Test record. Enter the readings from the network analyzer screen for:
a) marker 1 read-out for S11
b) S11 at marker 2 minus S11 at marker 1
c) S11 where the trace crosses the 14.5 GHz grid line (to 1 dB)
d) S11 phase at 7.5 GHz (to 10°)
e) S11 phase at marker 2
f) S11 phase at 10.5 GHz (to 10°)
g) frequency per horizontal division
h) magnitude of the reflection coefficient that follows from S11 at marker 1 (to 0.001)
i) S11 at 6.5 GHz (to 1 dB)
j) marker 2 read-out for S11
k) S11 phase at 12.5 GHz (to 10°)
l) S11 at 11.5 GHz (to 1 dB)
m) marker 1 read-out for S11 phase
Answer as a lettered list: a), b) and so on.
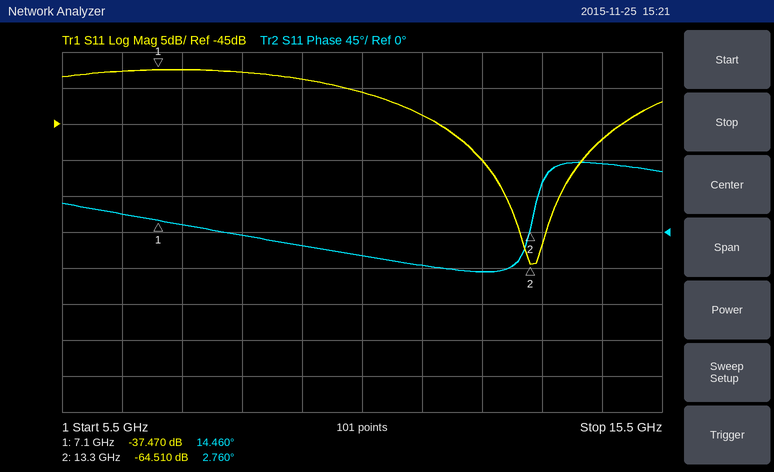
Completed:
a) -37.470 dB
b) -27.040 dB
c) -47 dB
d) 10°
e) 2.760°
f) -30°
g) 1 GHz
h) 0.013
i) -38 dB
j) -64.510 dB
k) -50°
l) -44 dB
m) 14.460°
